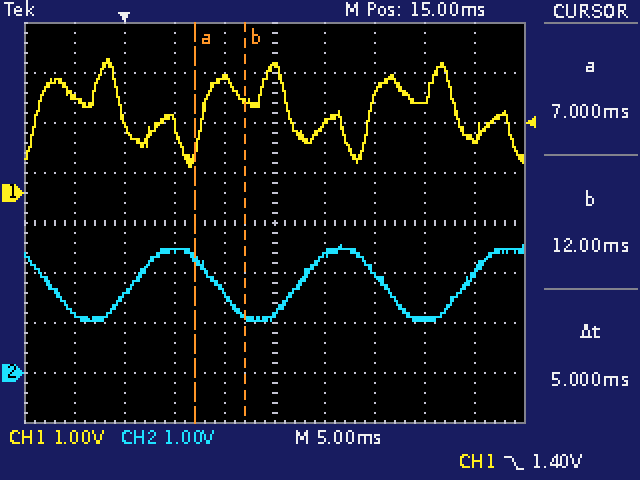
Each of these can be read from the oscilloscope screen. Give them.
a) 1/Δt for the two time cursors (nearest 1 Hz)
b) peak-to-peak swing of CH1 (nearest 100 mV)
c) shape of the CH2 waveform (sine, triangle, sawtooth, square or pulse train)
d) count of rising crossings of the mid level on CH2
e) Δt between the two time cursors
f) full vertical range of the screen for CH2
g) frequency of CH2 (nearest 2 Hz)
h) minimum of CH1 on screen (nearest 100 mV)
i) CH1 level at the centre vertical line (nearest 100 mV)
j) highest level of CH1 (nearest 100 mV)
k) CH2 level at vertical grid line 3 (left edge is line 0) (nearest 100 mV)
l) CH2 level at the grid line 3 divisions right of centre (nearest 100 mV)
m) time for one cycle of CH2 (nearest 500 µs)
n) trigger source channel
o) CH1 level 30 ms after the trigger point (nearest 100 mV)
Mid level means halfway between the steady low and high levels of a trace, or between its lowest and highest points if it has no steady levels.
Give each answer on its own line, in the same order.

200 Hz
2.2 V
sine
3
5 ms
8 V
60 Hz
500 mV
2.5 V
2.7 V
2.4 V
1.1 V
16.5 ms
CH1
1.9 V
